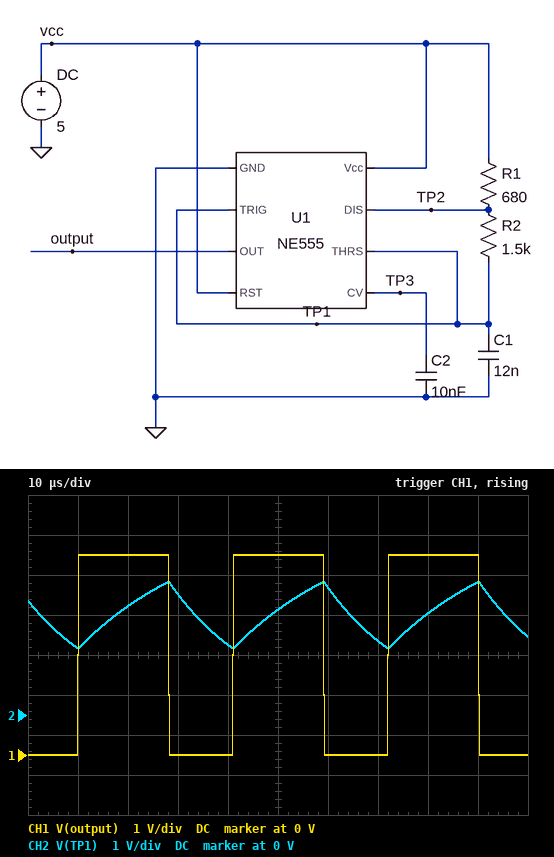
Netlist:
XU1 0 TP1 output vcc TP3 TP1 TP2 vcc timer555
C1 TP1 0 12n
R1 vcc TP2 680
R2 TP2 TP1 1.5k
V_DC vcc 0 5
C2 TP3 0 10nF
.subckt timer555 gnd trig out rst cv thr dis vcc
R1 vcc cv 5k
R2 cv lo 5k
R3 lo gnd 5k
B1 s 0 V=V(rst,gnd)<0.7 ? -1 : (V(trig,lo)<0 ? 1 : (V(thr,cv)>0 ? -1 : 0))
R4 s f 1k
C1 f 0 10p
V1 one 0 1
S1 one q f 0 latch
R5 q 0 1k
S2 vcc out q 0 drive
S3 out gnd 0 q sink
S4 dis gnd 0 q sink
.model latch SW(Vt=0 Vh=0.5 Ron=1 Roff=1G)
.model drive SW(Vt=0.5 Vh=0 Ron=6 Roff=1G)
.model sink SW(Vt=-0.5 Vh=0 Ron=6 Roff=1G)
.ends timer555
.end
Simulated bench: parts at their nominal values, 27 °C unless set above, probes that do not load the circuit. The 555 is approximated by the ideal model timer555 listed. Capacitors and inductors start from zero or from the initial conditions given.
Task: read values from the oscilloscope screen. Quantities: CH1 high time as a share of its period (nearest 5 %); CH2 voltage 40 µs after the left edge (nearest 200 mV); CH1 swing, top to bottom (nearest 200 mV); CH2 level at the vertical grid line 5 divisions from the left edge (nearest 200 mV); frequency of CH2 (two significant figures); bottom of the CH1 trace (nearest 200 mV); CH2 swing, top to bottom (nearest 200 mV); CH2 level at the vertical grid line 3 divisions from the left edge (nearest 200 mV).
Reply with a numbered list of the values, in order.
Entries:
1. 60 %
2. 1.8 V
3. 5.0 V
4. 2.6 V
5. 32 kHz
6. 0 V
7. 1.6 V
8. 3.0 V
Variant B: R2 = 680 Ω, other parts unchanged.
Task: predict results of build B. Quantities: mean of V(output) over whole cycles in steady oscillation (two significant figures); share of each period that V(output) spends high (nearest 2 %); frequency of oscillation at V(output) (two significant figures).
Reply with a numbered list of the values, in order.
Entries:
1. 3.3 V
2. 66 %
3. 58 kHz
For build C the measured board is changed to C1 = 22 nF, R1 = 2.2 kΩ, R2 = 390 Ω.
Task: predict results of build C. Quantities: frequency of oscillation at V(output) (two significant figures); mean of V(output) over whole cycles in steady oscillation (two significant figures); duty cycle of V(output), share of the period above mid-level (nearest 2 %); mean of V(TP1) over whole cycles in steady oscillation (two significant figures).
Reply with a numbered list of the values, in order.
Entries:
1. 22 kHz
2. 4.3 V
3. 86 %
4. 2.6 V
